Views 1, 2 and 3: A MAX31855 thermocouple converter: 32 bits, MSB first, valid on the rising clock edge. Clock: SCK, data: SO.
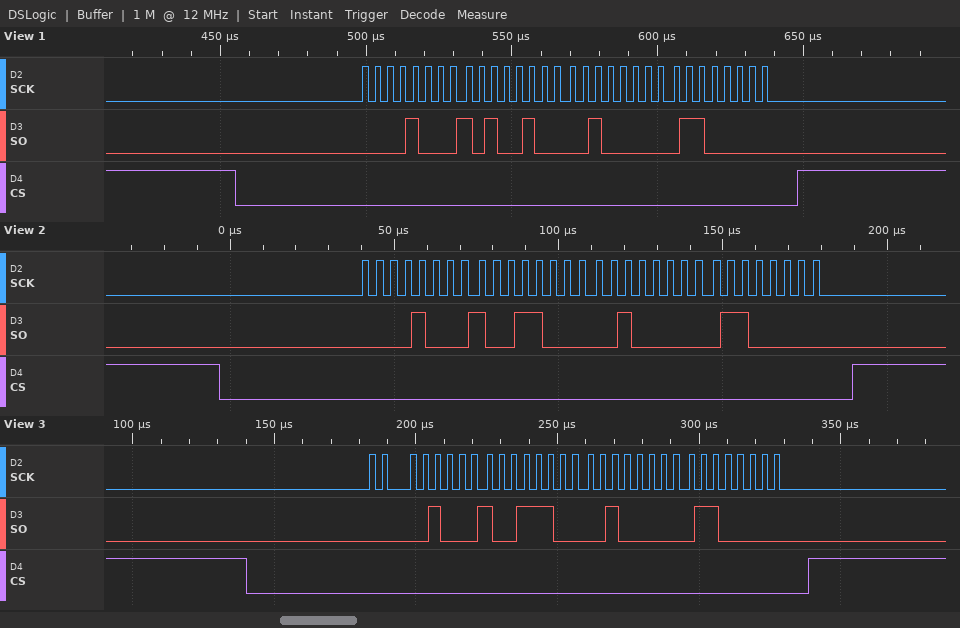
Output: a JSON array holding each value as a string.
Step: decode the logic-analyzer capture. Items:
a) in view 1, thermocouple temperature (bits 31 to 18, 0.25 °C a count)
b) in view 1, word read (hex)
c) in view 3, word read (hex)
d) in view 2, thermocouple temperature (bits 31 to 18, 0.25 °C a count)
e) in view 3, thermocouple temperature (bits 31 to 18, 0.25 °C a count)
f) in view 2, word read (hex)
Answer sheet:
["138.25 °C", "0x08A42060", "0x089C2060", "137.50 °C", "137.75 °C", "0x08982060"]
